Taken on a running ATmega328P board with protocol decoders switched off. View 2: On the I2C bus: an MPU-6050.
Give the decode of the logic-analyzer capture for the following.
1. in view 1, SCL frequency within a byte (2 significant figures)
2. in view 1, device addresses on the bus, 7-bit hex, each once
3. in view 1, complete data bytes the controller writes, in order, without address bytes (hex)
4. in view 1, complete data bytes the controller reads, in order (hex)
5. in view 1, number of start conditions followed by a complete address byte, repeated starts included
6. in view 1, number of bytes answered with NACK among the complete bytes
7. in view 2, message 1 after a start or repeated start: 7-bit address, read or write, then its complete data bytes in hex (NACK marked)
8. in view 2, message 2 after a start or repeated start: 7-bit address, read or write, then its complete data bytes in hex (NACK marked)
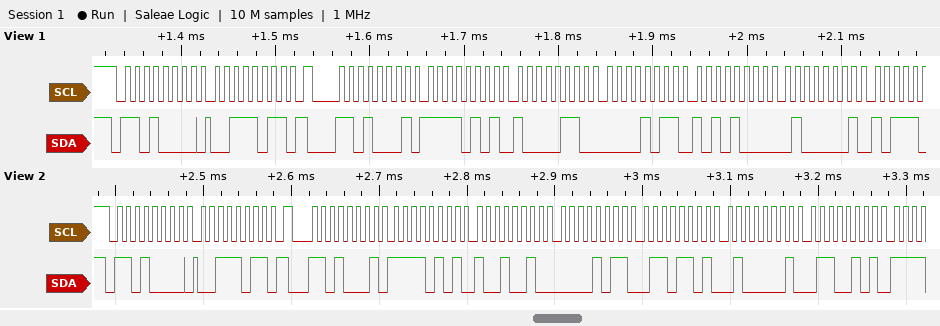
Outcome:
100 kHz
0x68
3B
F5 86 0B A8 41
2
0
0x68 write: 3B
0x68 read: F5 92 0B 6D 41 65
